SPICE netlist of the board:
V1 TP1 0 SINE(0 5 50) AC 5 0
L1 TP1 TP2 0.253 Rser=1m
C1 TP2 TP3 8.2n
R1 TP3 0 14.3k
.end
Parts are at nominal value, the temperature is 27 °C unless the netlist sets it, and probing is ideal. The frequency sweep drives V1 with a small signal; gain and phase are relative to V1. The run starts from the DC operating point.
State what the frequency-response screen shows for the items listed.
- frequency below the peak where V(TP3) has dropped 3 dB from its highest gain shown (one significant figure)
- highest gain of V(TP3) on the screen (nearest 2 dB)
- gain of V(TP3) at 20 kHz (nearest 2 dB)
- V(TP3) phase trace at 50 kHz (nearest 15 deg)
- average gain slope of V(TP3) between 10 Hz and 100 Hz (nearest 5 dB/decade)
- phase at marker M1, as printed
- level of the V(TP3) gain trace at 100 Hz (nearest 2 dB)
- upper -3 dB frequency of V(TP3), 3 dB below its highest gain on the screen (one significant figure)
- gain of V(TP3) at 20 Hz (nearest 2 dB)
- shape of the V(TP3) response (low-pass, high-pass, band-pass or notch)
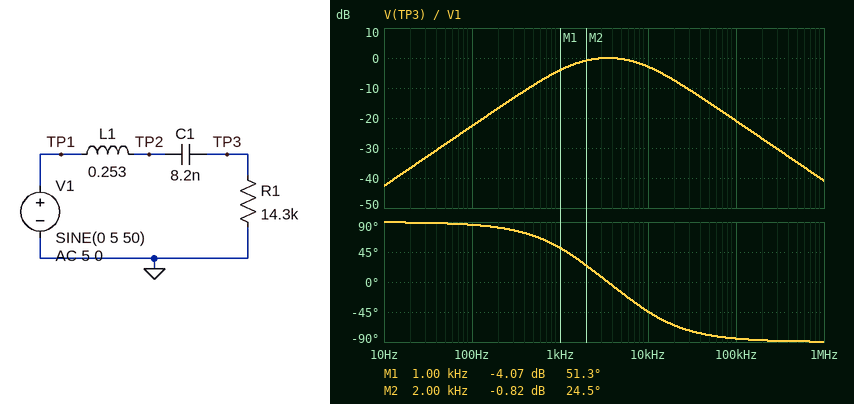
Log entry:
1 kHz
0 dB
-8 dB
-75 deg
20 dB/decade
51.3 deg
-22 dB
10 kHz
-36 dB
band-pass
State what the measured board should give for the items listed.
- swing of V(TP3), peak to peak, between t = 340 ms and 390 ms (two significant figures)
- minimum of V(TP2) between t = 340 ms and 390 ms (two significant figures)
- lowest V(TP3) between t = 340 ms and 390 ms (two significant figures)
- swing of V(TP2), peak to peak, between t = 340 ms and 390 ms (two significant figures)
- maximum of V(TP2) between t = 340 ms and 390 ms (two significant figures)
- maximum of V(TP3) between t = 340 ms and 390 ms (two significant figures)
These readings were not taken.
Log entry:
370 mV
-5.0 V
-180 mV
10 V
5.0 V
180 mV
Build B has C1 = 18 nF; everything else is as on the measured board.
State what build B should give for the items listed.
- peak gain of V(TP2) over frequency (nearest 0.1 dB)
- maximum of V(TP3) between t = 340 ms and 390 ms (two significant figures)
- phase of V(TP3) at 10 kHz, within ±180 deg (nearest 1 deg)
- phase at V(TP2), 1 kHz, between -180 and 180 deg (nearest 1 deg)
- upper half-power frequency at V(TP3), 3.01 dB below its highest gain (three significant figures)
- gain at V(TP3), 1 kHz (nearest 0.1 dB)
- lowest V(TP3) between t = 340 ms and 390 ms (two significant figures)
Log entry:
0.4 dB
400 mV
-46 deg
-5 deg
9.58 kHz
-1.0 dB
-400 mV
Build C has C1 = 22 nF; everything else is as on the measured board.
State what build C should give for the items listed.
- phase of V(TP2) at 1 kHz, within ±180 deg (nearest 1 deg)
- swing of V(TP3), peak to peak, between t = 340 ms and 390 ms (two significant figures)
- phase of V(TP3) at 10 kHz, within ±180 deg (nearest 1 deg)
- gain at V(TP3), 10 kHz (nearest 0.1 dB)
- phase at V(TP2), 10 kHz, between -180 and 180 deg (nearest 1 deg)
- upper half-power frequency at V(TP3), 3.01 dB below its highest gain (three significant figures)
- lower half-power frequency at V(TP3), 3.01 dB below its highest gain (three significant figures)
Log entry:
-5 deg
980 mV
-47 deg
-3.3 dB
-50 deg
9.48 kHz
480 Hz
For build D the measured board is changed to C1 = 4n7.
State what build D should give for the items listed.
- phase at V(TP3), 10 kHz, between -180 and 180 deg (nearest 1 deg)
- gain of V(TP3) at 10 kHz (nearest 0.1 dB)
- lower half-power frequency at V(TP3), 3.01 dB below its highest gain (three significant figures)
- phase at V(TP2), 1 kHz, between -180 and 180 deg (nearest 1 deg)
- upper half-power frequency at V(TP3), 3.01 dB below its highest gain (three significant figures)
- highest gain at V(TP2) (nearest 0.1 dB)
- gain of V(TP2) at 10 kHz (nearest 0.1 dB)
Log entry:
-41 deg
-2.5 dB
1.95 kHz
-1 deg
10.9 kHz
1.3 dB
-2.2 dB
